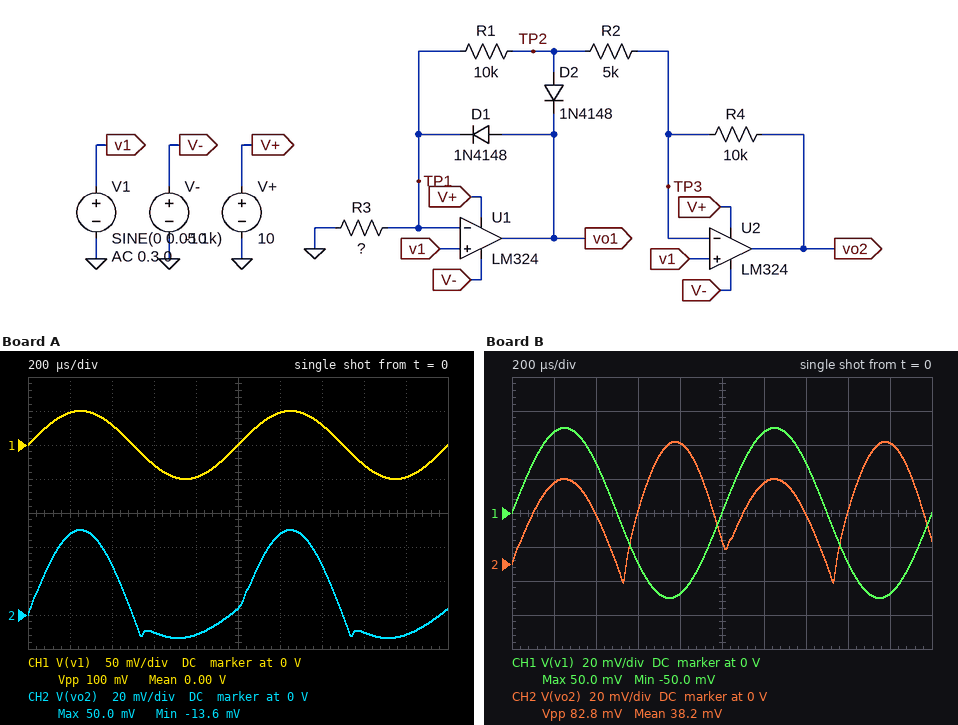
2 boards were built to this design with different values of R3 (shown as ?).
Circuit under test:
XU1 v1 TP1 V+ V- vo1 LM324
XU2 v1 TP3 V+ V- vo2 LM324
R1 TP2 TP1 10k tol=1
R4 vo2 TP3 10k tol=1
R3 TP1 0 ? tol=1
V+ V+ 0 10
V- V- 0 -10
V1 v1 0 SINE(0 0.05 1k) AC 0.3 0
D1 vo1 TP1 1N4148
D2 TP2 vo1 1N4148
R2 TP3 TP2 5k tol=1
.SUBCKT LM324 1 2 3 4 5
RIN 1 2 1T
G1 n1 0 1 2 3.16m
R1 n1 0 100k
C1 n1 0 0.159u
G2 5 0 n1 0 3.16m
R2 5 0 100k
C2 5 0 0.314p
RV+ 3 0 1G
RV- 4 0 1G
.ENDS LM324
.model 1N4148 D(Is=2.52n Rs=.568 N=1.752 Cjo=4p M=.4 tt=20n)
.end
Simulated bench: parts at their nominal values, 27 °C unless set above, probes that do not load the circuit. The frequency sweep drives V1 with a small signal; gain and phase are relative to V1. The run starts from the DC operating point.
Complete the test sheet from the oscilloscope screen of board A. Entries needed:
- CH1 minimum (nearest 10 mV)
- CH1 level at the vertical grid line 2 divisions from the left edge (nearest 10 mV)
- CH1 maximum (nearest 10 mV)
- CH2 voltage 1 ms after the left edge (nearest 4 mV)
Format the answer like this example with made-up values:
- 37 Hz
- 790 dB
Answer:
- -50 mV
- 30 mV
- 50 mV
- 4 mV
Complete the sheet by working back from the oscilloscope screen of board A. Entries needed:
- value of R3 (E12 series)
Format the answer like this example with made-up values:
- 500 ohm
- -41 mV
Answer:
- 27 kΩ
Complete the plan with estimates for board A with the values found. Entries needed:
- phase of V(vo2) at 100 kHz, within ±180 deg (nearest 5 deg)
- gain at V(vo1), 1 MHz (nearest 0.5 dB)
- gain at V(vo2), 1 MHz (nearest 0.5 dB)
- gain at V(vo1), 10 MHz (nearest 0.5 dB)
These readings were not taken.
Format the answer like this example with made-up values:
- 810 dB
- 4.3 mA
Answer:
- -15 deg
- -9.0 dB
- -7.0 dB
- -31.5 dB
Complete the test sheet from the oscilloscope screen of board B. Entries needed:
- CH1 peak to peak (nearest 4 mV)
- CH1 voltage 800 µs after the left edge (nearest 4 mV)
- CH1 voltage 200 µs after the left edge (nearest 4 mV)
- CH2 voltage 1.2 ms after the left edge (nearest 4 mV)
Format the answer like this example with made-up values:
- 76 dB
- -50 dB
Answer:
- 100 mV
- -48 mV
- 48 mV
- 48 mV
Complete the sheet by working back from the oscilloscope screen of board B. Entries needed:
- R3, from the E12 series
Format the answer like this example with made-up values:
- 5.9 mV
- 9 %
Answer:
- 8.2 kΩ
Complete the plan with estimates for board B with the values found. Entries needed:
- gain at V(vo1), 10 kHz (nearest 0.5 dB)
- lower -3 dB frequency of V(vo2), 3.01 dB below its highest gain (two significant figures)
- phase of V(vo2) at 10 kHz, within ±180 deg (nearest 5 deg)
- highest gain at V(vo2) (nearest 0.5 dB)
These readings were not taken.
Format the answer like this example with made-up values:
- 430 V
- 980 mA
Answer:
- 34.5 dB
- 300 Hz
- 0 deg
- 2.0 dB
